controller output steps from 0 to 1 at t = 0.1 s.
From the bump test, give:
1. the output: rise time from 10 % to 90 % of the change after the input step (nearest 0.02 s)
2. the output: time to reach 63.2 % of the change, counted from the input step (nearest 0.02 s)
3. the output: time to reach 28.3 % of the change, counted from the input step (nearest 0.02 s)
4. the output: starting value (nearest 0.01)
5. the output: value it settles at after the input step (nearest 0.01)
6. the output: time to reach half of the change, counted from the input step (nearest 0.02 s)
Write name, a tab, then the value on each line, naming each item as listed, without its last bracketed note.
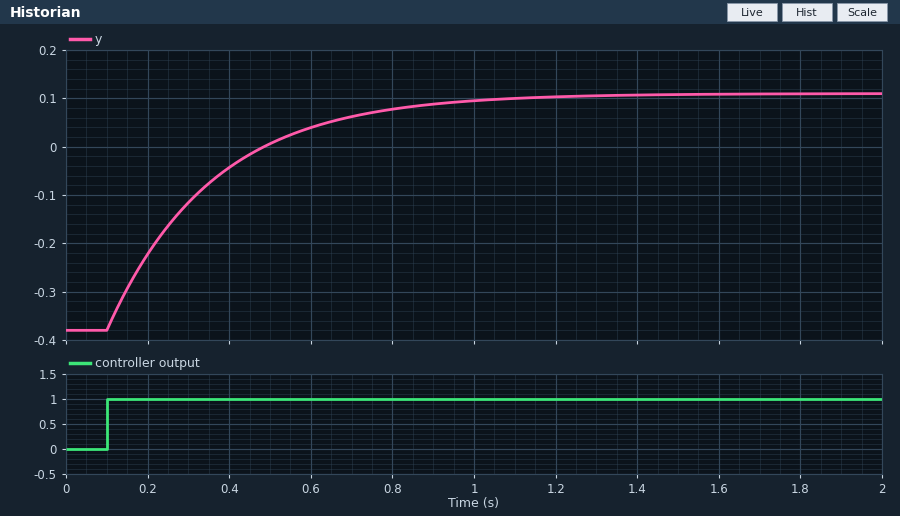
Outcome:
the output: rise time from 10 % to 90 % of the change after the input step	0.56 s
the output: time to reach 63.2 % of the change, counted from the input step	0.26 s
the output: time to reach 28.3 % of the change, counted from the input step	0.08 s
the output: starting value	-0.38
the output: value it settles at after the input step	0.11
the output: time to reach half of the change, counted from the input step	0.18 s
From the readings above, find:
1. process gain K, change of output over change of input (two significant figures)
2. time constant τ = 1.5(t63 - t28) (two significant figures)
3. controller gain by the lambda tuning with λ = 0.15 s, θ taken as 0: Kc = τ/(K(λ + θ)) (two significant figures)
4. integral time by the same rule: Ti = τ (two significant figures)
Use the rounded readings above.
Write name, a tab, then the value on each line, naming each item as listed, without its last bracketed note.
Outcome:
process gain K, change of output over change of input	0.49
time constant τ = 1.5(t63 - t28)	0.27 s
controller gain by the lambda tuning with λ = 0.15 s, θ taken as 0: Kc = τ/(K(λ + θ))	3.7
integral time by the same rule: Ti = τ	0.27 s
